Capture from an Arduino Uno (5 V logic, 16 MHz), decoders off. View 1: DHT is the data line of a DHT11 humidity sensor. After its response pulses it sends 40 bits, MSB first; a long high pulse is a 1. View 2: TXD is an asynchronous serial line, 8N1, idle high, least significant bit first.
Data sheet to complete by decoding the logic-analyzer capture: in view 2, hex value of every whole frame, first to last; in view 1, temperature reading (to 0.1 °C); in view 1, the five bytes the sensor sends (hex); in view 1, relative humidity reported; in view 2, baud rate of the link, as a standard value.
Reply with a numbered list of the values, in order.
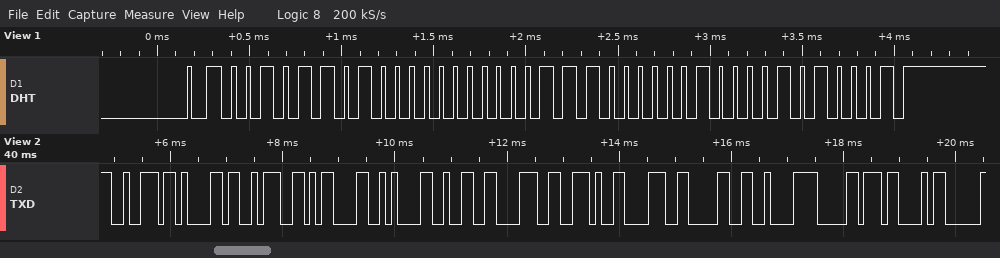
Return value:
1. 72 61 3A 0D 0A 32 38 2E 38 30 C2 B0 43
2. 28.8 °C
3. 2D 00 1C 08 51
4. 45 %
5. 9600 baud
